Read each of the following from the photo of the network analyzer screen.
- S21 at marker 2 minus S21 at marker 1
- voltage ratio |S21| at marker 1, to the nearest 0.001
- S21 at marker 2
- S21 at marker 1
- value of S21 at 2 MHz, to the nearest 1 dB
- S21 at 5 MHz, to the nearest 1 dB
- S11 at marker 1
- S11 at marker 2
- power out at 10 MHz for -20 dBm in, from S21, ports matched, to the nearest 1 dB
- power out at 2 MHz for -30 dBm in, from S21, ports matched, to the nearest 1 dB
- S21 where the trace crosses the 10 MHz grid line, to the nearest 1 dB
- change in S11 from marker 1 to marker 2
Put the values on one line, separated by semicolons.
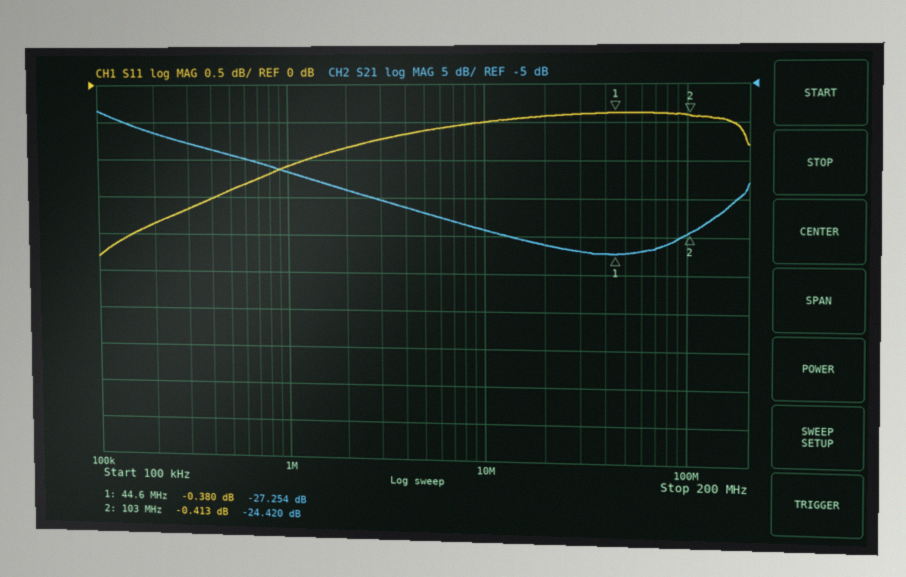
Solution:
2.834 dB; 0.043; -24.420 dB; -27.254 dB; -19 dB; -22 dB; -0.380 dB; -0.413 dB; -44 dBm; -49 dBm; -24 dB; -0.033 dB
